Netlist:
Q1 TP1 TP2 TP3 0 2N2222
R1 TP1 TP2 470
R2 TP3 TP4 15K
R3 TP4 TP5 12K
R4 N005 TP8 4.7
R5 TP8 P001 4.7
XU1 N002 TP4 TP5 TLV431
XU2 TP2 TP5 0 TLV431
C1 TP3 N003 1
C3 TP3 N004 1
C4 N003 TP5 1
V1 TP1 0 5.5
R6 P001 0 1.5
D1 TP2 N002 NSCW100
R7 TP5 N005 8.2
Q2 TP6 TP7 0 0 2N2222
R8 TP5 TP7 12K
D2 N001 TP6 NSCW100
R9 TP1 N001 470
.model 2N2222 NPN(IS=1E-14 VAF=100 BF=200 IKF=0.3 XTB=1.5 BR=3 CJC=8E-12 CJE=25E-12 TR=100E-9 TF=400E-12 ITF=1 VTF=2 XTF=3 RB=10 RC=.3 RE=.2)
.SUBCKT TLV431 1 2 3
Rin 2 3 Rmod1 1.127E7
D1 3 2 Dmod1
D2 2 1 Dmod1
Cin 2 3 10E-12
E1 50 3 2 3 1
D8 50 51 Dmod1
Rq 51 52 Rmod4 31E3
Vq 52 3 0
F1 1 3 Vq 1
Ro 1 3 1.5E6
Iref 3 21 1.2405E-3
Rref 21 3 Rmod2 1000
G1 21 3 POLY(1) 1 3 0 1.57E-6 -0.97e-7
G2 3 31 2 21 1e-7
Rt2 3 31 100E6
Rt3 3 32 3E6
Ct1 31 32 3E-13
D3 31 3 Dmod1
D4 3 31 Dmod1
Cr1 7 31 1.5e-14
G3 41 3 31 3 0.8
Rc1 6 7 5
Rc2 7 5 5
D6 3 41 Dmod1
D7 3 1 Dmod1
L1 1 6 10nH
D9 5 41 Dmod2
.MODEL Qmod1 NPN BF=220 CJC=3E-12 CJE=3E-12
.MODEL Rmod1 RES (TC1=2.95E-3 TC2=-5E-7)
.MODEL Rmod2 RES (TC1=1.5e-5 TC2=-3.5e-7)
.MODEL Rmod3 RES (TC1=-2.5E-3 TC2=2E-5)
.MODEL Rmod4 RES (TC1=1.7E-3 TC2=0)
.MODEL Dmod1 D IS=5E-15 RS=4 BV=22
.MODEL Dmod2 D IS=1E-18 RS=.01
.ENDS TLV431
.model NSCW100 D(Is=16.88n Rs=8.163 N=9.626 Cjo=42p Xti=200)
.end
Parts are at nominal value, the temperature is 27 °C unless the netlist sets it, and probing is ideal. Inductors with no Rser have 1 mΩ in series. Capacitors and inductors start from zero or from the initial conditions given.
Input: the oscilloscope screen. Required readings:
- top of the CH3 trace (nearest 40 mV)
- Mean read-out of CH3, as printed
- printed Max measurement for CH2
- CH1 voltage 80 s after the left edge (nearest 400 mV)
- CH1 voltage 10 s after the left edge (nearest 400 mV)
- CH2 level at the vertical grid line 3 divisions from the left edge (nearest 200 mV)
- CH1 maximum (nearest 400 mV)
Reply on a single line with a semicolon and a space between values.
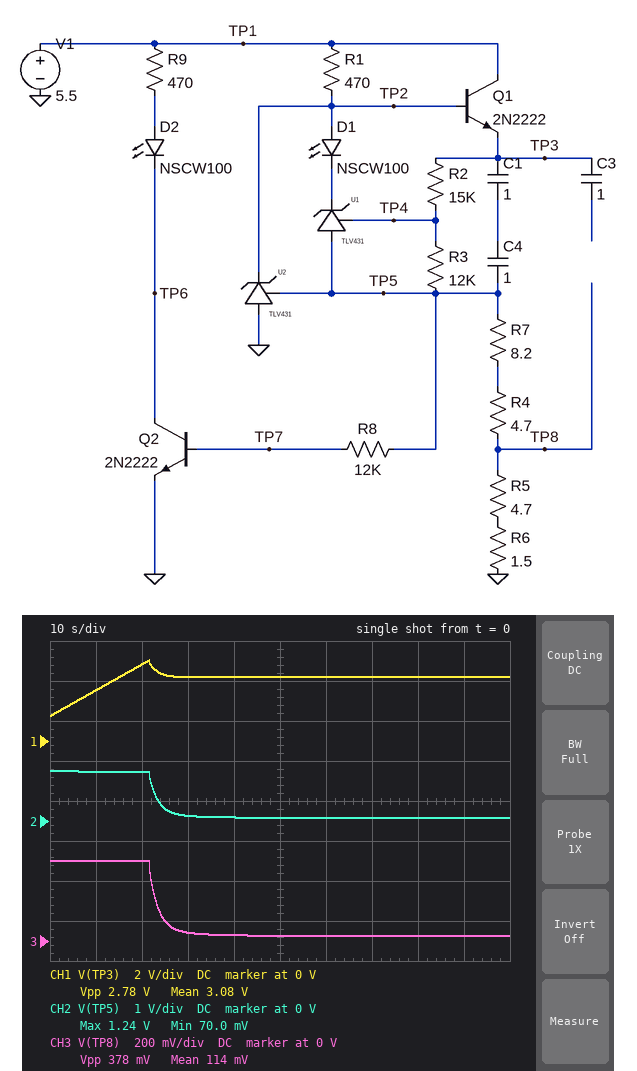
400 mV; 114 mV; 1.24 V; 3.2 V; 2.4 V; 200 mV; 4.0 V
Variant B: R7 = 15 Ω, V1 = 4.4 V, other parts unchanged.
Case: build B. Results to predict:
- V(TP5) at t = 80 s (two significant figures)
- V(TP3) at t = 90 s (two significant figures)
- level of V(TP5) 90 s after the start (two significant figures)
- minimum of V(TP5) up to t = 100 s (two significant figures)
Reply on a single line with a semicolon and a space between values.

52 mV; 3.0 V; 51 mV; 50 mV
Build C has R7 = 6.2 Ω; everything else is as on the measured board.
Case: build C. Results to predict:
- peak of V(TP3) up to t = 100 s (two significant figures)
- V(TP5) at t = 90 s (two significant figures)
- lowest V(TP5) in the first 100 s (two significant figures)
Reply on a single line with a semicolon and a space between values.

4.0 V; 66 mV; 65 mV
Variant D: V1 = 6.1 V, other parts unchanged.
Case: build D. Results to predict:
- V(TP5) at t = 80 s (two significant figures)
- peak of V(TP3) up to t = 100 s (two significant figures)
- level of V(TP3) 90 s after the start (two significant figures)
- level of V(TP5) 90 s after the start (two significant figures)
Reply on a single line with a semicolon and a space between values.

95 mV; 4.1 V; 3.3 V; 94 mV
